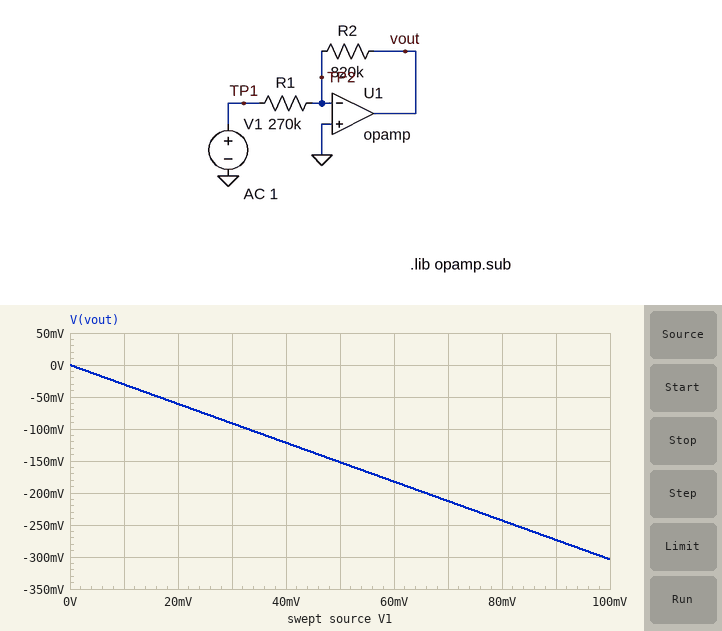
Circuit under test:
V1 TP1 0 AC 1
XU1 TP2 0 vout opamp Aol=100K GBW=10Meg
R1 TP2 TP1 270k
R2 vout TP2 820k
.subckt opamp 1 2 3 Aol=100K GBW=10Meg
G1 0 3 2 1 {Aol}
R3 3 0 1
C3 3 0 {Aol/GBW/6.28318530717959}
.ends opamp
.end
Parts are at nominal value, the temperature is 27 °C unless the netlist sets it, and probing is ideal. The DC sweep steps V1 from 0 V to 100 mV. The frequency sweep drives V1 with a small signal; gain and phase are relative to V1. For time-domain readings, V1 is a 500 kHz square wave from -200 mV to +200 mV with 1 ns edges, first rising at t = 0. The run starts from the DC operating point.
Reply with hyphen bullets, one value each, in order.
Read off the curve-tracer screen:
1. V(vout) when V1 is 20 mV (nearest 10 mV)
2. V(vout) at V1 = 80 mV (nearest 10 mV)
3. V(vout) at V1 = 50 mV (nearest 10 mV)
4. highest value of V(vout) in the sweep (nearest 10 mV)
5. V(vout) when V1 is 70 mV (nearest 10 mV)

- -60 mV
- -240 mV
- -150 mV
- 0 V
- -210 mV
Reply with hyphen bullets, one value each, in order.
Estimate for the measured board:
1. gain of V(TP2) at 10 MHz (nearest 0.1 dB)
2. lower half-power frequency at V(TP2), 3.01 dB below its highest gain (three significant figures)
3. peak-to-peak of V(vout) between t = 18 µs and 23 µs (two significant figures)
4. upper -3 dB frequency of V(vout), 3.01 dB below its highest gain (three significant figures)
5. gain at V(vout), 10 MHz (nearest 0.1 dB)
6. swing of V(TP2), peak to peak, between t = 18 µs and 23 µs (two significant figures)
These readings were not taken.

- -2.7 dB
- 2.48 MHz
- 1.2 V
- 2.48 MHz
- -2.7 dB
- 600 mV
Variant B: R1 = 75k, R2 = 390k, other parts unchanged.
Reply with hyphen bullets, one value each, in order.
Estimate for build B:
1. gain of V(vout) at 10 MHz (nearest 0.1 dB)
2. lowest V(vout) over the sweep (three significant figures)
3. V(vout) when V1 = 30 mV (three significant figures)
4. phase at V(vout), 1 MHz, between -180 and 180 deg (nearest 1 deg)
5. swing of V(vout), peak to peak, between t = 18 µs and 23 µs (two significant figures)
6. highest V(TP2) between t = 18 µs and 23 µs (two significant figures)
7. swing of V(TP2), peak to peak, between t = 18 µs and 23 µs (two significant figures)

- -1.6 dB
- -520 mV
- -156 mV
- 148 deg
- 2.1 V
- 330 mV
- 670 mV
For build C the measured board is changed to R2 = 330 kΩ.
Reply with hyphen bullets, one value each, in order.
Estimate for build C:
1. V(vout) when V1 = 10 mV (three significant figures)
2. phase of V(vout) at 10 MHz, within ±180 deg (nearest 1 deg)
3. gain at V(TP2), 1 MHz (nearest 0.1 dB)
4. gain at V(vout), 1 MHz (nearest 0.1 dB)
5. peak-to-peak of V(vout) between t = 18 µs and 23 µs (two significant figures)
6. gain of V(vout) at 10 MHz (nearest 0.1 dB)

- -12.2 mV
- 114 deg
- -18.5 dB
- 1.5 dB
- 490 mV
- -6.0 dB
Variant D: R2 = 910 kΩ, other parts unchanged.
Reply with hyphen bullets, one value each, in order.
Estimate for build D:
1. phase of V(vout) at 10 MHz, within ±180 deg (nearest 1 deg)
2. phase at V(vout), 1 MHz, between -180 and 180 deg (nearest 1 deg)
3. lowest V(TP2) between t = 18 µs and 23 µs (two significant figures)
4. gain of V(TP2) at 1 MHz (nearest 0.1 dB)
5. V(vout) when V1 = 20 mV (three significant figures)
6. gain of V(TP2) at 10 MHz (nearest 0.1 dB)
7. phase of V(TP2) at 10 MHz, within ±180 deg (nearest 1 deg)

- 103 deg
- 156 deg
- -310 mV
- -10.2 dB
- -67.4 mV
- -2.5 dB
- 13 deg
